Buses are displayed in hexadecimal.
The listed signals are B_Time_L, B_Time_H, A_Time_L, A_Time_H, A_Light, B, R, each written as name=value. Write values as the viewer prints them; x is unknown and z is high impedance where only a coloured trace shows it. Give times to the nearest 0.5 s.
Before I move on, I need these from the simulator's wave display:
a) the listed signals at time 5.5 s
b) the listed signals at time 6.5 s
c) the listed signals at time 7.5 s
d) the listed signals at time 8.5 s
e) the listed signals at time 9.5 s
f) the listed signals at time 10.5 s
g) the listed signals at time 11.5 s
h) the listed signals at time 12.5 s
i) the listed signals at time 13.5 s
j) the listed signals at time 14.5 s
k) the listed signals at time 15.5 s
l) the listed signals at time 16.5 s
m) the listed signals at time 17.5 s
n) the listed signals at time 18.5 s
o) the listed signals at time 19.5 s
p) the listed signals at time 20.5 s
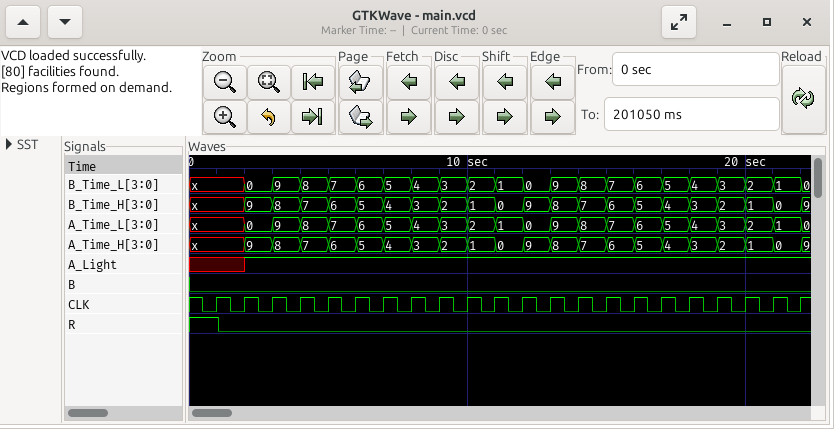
B_Time_L=7, B_Time_H=6, A_Time_L=7, A_Time_H=6, A_Light=1, B=0, R=0
B_Time_L=6, B_Time_H=5, A_Time_L=6, A_Time_H=5, A_Light=1, B=0, R=0
B_Time_L=5, B_Time_H=4, A_Time_L=5, A_Time_H=4, A_Light=1, B=0, R=0
B_Time_L=4, B_Time_H=3, A_Time_L=4, A_Time_H=3, A_Light=1, B=0, R=0
B_Time_L=3, B_Time_H=2, A_Time_L=3, A_Time_H=2, A_Light=1, B=0, R=0
B_Time_L=2, B_Time_H=1, A_Time_L=2, A_Time_H=1, A_Light=1, B=0, R=0
B_Time_L=1, B_Time_H=0, A_Time_L=1, A_Time_H=0, A_Light=1, B=0, R=0
B_Time_L=0, B_Time_H=9, A_Time_L=0, A_Time_H=9, A_Light=1, B=0, R=0
B_Time_L=9, B_Time_H=8, A_Time_L=9, A_Time_H=8, A_Light=1, B=0, R=0
B_Time_L=8, B_Time_H=7, A_Time_L=8, A_Time_H=7, A_Light=1, B=0, R=0
B_Time_L=7, B_Time_H=6, A_Time_L=7, A_Time_H=6, A_Light=1, B=0, R=0
B_Time_L=6, B_Time_H=5, A_Time_L=6, A_Time_H=5, A_Light=1, B=0, R=0
B_Time_L=5, B_Time_H=4, A_Time_L=5, A_Time_H=4, A_Light=1, B=0, R=0
B_Time_L=4, B_Time_H=3, A_Time_L=4, A_Time_H=3, A_Light=1, B=0, R=0
B_Time_L=3, B_Time_H=2, A_Time_L=3, A_Time_H=2, A_Light=1, B=0, R=0
B_Time_L=2, B_Time_H=1, A_Time_L=2, A_Time_H=1, A_Light=1, B=0, R=0
